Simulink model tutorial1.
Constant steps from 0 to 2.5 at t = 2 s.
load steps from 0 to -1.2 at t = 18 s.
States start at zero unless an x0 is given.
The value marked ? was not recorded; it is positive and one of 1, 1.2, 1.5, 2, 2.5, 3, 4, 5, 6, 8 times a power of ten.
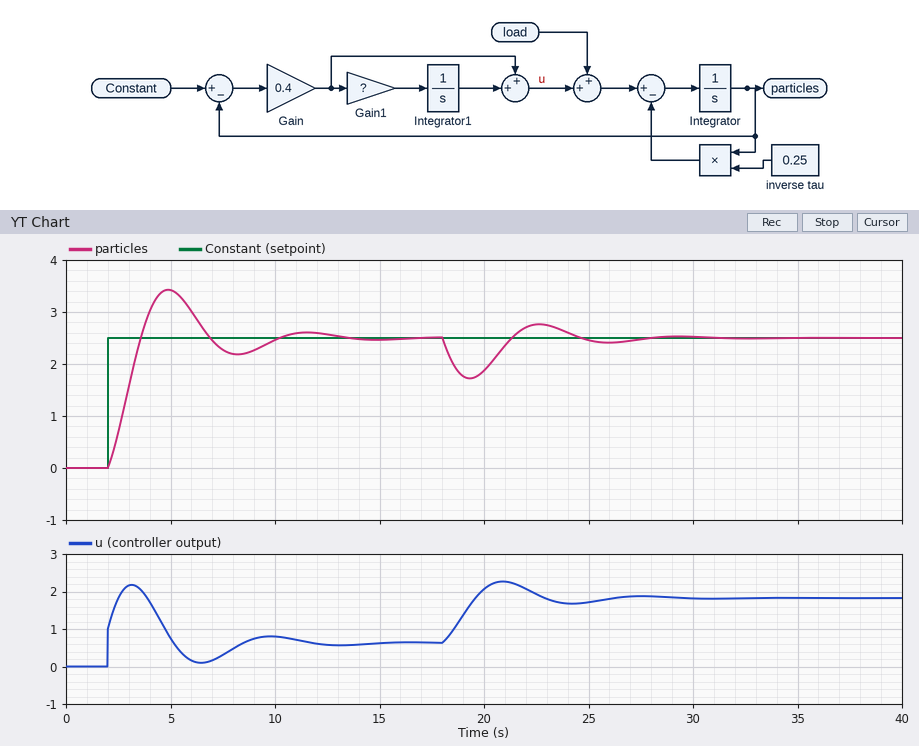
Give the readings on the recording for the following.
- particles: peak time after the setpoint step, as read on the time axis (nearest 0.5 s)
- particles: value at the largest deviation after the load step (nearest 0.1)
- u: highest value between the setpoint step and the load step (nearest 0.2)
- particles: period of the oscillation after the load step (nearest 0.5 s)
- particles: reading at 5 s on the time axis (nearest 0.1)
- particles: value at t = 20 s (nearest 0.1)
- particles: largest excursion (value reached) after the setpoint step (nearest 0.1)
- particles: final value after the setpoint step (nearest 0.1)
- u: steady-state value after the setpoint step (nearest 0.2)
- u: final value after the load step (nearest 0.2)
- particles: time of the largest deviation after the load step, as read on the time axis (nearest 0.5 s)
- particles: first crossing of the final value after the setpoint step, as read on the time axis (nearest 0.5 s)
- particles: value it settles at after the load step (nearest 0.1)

5.0 s
1.7
2.2
6.5 s
3.4
1.9
3.4
2.5
0.6
1.8
19.5 s
3.5 s
2.5
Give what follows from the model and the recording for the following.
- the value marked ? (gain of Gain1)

2.5
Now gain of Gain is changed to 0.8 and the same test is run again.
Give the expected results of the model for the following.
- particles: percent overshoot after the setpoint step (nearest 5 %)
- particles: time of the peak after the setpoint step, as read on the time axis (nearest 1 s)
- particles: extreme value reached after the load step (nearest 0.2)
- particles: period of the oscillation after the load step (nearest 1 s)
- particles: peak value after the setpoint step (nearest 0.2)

35 %
4 s
2.0
5 s
3.4
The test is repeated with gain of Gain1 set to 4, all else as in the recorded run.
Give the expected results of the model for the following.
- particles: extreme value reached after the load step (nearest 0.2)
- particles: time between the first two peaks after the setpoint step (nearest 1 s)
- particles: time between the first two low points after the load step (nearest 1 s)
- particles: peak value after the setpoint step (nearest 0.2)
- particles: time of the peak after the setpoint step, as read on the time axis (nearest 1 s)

1.8
5 s
5 s
3.6
4 s
